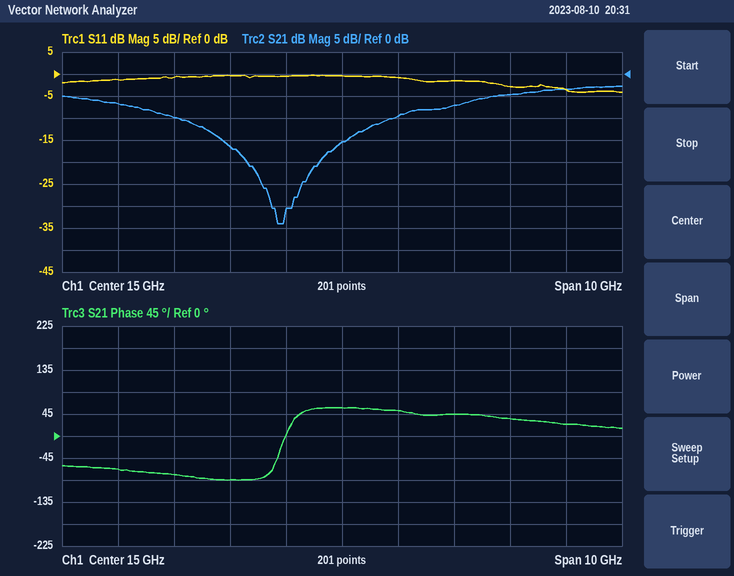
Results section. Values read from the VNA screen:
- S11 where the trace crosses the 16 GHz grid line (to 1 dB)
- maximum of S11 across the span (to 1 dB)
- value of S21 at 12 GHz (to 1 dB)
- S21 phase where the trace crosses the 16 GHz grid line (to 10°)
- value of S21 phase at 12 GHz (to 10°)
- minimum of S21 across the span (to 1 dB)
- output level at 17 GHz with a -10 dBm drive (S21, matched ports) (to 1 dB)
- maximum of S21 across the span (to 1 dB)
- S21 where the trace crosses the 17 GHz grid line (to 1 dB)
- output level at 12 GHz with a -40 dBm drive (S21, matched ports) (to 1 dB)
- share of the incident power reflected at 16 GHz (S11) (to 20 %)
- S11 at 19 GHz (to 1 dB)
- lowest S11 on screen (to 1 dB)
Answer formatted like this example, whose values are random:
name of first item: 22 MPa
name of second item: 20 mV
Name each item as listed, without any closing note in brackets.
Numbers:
S11 where the trace crosses the 16 GHz grid line: -1 dB
maximum of S11 across the span: 0 dB
value of S21 at 12 GHz: -10 dB
S21 phase where the trace crosses the 16 GHz grid line: 50°
value of S21 phase at 12 GHz: -80°
minimum of S21 across the span: -34 dB
output level at 17 GHz with a -10 dBm drive (S21, matched ports): -17 dBm
maximum of S21 across the span: -3 dB
S21 where the trace crosses the 17 GHz grid line: -7 dB
output level at 12 GHz with a -40 dBm drive (S21, matched ports): -50 dBm
share of the incident power reflected at 16 GHz (S11): 80 %
S11 at 19 GHz: -4 dB
lowest S11 on screen: -4 dB
